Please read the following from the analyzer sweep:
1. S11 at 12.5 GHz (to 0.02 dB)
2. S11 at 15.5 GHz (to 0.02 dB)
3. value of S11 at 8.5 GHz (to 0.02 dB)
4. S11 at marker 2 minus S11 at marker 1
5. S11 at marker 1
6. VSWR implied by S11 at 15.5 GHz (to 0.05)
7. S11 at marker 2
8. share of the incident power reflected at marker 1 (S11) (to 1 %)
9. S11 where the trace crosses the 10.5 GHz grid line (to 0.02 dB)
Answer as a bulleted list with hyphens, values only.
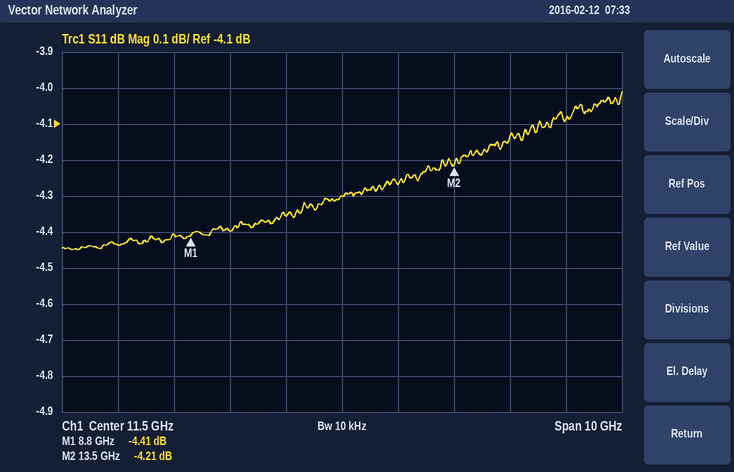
- -4.26 dB
- -4.08 dB
- -4.40 dB
- 0.20 dB
- -4.41 dB
- 4.35
- -4.21 dB
- 36 %
- -4.36 dB
